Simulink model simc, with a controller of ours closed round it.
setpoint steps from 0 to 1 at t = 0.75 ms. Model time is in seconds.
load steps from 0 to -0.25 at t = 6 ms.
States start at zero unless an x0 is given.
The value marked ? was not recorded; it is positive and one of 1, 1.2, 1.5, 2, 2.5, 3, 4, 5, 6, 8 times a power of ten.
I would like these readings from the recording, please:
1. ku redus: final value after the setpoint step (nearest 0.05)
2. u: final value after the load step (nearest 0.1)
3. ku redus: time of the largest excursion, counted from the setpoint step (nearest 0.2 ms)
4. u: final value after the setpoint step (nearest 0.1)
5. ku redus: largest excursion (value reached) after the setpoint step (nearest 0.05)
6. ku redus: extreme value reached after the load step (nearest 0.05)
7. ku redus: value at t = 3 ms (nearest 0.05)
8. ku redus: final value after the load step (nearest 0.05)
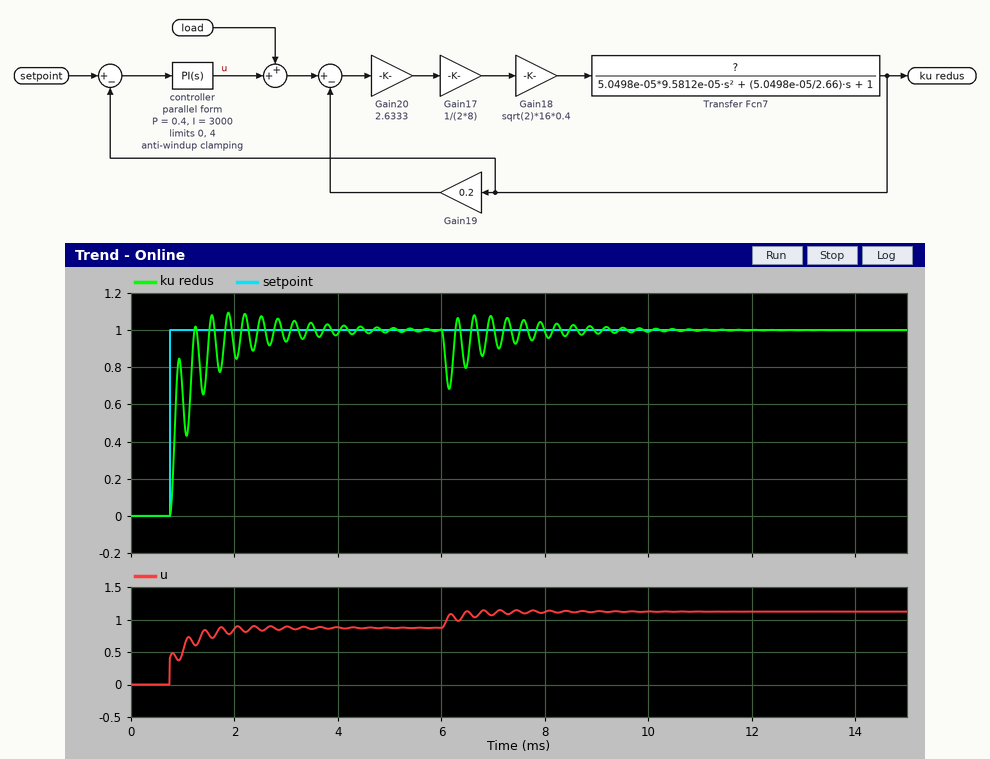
1.00
1.1
1.2 ms
0.9
1.10
0.70
0.95
1.00
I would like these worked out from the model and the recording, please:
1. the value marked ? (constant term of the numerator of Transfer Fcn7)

1
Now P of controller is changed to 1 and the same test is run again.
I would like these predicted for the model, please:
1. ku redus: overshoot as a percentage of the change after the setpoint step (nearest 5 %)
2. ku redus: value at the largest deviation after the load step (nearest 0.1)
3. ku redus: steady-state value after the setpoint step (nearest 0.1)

10 %
0.8
1.0
